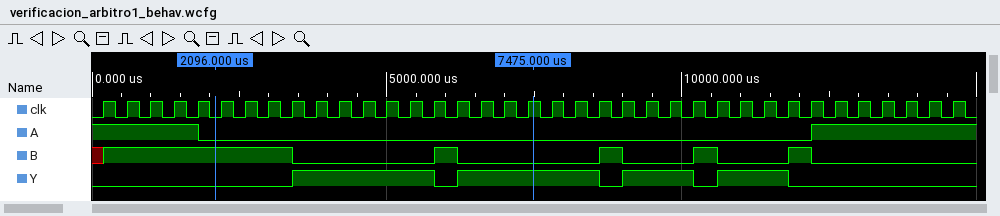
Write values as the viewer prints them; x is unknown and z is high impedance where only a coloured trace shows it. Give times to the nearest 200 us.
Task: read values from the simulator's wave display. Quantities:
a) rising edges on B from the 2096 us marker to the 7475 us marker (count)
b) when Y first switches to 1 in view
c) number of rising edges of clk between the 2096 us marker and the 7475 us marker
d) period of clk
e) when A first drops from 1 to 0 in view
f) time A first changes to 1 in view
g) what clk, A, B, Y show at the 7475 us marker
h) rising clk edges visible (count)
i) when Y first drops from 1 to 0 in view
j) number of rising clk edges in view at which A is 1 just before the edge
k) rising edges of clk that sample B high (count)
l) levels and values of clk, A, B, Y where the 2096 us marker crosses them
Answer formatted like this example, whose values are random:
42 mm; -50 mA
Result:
1; 3400 us; 14; 400 us; 1800 us; 12200 us; clk=1, A=0, B=0, Y=1; 37; 5800 us; 11; 12; clk=0, A=0, B=1, Y=0
